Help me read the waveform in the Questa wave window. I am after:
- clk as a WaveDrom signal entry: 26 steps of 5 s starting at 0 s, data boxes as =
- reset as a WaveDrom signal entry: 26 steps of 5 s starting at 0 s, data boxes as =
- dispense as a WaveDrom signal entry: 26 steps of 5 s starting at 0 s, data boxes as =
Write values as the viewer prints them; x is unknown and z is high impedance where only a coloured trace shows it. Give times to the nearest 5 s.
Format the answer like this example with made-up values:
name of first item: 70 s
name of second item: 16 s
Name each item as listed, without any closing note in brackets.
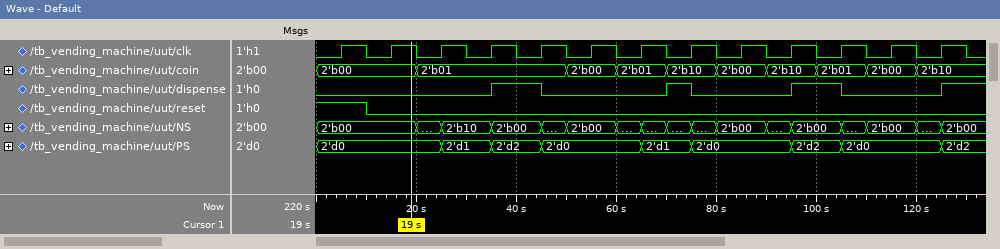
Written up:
clk as a WaveDrom signal entry: 26 steps of 5 s starting at 0 s, data boxes as =: {name: 'clk', wave: '01010101010101010101010101'}
reset as a WaveDrom signal entry: 26 steps of 5 s starting at 0 s, data boxes as =: {name: 'reset', wave: '1.0.......................'}
dispense as a WaveDrom signal entry: 26 steps of 5 s starting at 0 s, data boxes as =: {name: 'dispense', wave: '0......1.0....10...1.0...1'}
